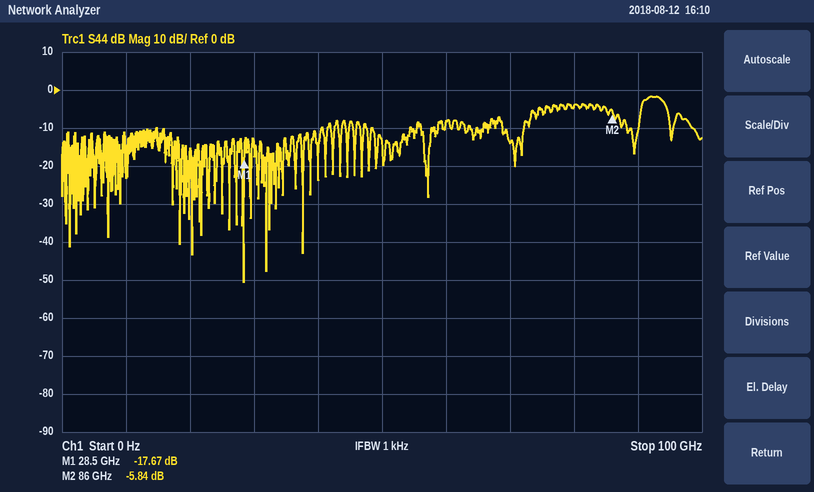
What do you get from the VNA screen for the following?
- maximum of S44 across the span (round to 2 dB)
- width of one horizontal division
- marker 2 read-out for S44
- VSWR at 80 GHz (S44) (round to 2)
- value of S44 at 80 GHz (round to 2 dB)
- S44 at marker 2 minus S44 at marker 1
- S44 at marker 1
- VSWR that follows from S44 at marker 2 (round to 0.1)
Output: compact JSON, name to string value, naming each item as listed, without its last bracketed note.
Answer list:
{"maximum of S44 across the span": "-2 dB", "width of one horizontal division": "10 GHz", "marker 2 read-out for S44": "-5.84 dB", "VSWR at 80 GHz (S44)": "4", "value of S44 at 80 GHz": "-4 dB", "S44 at marker 2 minus S44 at marker 1": "11.83 dB", "S44 at marker 1": "-17.67 dB", "VSWR that follows from S44 at marker 2": "3.1"}
